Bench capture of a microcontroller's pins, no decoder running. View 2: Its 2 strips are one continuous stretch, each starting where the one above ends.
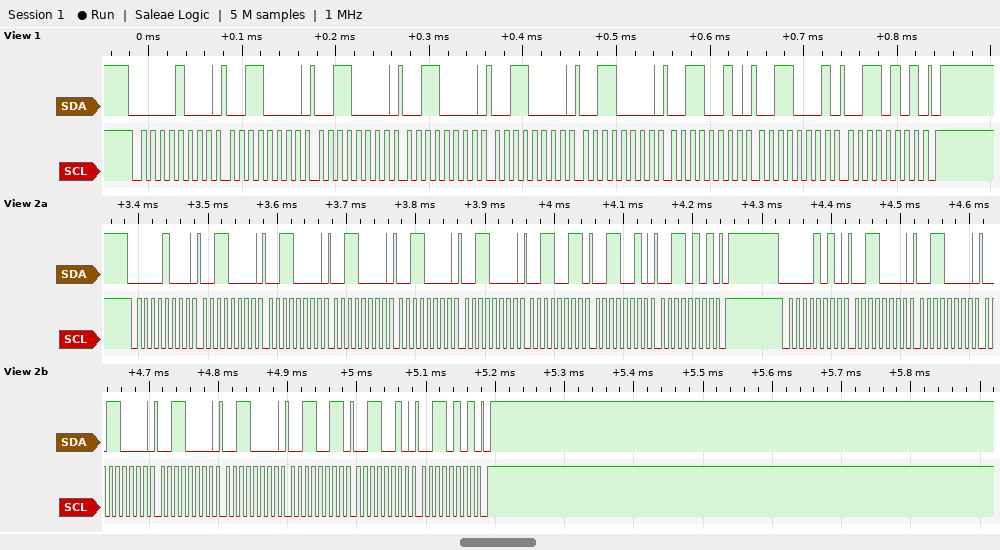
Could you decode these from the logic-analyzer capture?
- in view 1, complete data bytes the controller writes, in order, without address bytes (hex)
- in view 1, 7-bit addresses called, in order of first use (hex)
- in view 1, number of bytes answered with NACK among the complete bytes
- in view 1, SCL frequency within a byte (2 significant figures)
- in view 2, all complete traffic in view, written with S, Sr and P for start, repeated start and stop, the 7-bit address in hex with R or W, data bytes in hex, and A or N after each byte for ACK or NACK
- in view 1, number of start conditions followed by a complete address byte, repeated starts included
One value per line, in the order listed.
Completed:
30 30 30 30 30 32 31 35
0x04
0
100 kHz
S 04W A 30 A 30 A 30 A 30 A 30 A 33 A 32 A 35 A P S 05W A 30 A 30 A 30 A 30 A 30 A 33 A 32 A 35 A P
1
